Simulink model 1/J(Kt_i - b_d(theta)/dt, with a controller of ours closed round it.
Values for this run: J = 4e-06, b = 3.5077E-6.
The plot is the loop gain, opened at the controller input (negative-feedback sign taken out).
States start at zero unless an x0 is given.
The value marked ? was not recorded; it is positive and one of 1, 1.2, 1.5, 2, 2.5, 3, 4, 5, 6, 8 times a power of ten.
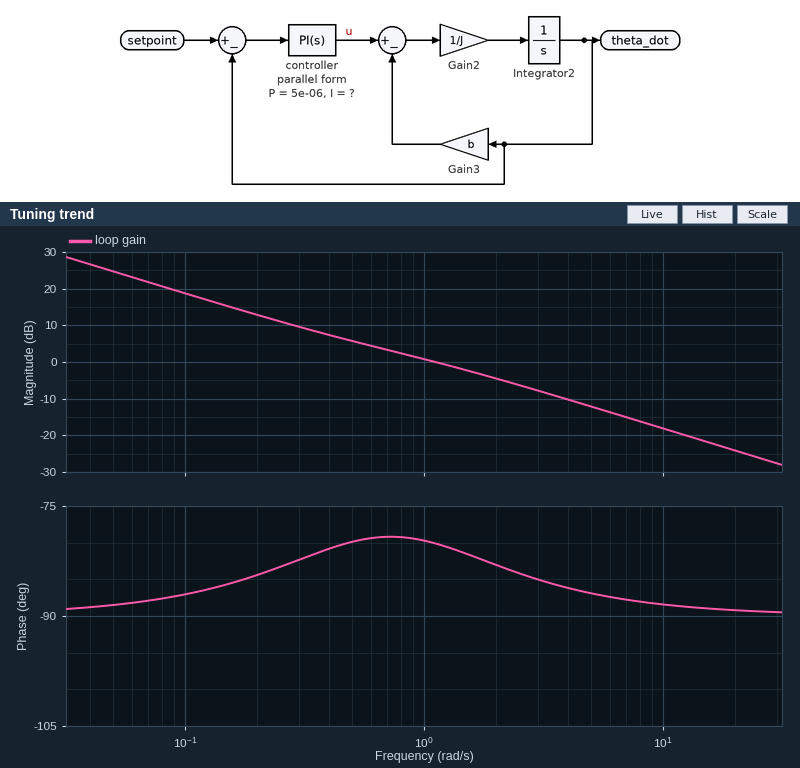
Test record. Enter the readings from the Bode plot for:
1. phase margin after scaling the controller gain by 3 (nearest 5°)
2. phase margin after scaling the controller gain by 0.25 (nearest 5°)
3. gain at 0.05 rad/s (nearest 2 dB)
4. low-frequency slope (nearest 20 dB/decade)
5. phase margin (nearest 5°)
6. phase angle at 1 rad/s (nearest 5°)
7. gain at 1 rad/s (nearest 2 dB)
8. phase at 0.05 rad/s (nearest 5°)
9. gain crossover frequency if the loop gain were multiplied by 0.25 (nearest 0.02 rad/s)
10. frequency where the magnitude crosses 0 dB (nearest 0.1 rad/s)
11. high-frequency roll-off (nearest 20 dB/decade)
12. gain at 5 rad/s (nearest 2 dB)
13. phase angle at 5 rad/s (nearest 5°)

95°
95°
24 dB
-20 dB/decade
100°
-80°
0 dB
-90°
0.22 rad/s
1.1 rad/s
-20 dB/decade
-12 dB
-85°
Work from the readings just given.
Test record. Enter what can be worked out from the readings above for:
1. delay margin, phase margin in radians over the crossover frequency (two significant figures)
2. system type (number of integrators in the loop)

1.6 s
1
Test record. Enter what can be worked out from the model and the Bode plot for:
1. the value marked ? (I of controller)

3e-06
